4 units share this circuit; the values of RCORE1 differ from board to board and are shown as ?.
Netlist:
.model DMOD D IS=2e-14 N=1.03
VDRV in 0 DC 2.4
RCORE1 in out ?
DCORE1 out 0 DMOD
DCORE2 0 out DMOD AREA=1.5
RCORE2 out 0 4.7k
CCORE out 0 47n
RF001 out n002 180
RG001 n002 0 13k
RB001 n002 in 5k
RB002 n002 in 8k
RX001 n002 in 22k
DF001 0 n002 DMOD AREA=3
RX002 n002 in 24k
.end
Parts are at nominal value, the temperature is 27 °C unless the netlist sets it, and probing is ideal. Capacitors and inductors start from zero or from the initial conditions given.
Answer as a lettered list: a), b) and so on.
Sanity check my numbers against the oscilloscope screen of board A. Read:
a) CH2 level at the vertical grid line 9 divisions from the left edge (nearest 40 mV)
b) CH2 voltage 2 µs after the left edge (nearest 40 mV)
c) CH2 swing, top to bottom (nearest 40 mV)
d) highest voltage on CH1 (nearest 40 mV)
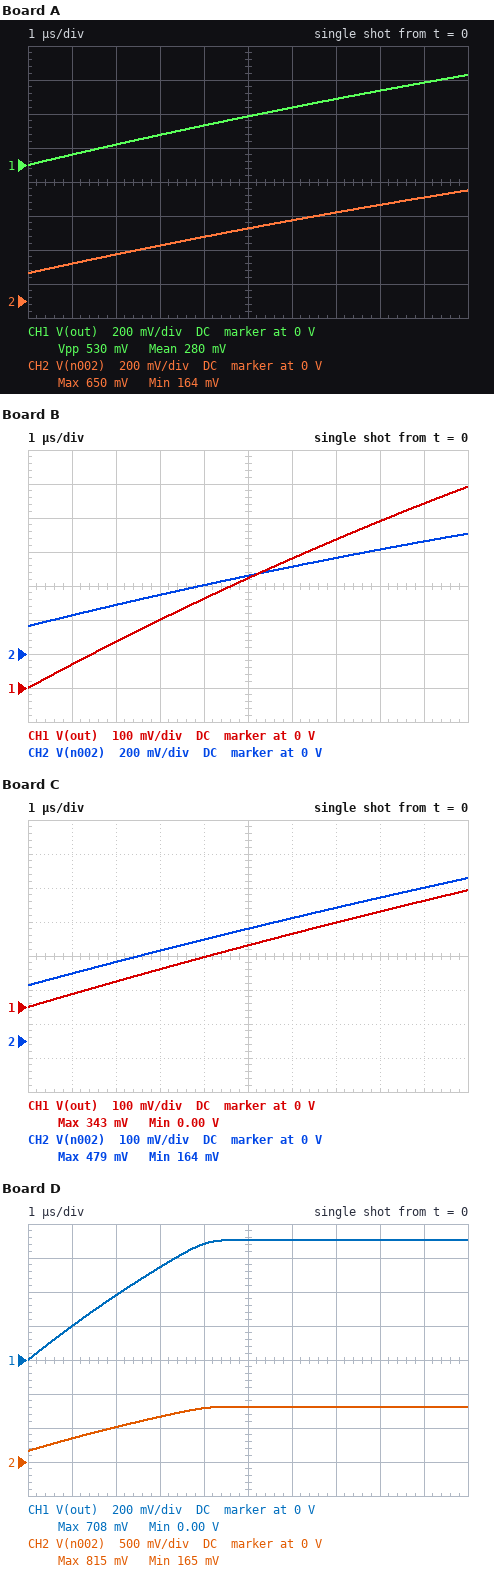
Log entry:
a) 600 mV
b) 280 mV
c) 480 mV
d) 520 mV
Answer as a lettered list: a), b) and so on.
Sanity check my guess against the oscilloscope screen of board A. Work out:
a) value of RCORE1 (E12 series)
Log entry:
a) 1.2 kΩ
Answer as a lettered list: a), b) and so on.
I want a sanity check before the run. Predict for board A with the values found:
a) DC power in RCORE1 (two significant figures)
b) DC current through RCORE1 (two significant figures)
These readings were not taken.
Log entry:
a) 2.5 mW
b) 1.4 mA
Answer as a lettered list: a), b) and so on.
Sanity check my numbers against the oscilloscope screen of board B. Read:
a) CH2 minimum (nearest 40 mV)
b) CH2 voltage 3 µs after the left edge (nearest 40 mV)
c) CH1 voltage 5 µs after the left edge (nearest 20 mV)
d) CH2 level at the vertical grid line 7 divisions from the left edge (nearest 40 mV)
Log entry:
a) 160 mV
b) 360 mV
c) 320 mV
d) 560 mV
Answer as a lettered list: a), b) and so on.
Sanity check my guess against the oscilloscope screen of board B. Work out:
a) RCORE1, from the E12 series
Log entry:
a) 1 kΩ
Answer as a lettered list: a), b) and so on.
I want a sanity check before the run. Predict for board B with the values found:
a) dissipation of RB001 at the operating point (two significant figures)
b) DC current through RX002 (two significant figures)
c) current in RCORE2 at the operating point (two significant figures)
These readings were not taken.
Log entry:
a) 520 µW
b) 67 µA
c) 140 µA
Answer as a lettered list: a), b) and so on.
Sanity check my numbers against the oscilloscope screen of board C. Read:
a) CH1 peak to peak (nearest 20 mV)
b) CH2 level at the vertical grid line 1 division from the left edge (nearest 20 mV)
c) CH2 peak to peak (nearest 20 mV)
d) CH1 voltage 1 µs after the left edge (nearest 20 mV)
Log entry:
a) 340 mV
b) 200 mV
c) 320 mV
d) 40 mV
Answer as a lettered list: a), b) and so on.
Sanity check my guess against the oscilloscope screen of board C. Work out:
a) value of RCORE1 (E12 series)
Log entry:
a) 2.7 kΩ
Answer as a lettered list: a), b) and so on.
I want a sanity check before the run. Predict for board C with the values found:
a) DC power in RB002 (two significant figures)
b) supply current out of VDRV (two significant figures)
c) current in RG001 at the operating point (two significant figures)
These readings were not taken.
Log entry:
a) 330 µW
b) 1.3 mA
c) 59 µA
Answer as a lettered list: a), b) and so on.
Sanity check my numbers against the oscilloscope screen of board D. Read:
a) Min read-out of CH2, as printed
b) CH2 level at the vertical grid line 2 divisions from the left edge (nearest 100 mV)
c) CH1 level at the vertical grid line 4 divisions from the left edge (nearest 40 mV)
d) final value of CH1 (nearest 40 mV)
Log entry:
a) 165 mV
b) 500 mV
c) 680 mV
d) 720 mV
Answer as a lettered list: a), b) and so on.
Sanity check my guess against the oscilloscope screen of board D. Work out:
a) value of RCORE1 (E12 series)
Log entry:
a) 270 Ω
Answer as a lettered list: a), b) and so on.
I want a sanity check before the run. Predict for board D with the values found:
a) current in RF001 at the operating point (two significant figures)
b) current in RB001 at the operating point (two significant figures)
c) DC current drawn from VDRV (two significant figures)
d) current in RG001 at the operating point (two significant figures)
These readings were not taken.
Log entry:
a) 590 µA
b) 320 µA
c) 6.9 mA
d) 63 µA
